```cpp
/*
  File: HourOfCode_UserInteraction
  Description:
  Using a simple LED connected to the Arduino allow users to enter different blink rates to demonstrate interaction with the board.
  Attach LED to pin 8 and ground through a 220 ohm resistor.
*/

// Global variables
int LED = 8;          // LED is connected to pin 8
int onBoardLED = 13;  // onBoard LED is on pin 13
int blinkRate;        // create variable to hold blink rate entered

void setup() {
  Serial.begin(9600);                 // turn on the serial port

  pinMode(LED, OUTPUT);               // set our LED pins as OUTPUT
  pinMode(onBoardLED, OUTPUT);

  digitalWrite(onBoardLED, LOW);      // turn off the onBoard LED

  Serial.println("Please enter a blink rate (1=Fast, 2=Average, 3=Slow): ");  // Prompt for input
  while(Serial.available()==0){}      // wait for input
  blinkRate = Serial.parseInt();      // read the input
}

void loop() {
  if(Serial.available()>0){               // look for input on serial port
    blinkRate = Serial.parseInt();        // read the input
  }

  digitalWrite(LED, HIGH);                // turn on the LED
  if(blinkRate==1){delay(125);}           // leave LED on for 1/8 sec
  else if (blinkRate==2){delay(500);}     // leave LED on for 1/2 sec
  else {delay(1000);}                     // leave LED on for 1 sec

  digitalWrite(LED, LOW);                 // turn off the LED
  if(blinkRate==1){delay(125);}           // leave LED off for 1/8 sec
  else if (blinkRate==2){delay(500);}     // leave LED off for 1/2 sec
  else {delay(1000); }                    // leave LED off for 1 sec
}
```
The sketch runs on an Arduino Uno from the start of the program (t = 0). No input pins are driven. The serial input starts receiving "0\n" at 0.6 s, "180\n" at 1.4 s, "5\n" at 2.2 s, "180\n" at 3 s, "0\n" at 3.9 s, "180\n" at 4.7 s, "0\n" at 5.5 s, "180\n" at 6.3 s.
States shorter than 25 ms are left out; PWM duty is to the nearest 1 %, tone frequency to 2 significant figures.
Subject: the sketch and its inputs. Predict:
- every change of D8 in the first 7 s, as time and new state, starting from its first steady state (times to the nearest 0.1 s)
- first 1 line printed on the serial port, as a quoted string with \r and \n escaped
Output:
0 s low; 1.4 s high; 2.4 s low; 3.4 s high; 4.4 s low; 5.4 s high; 6.4 s low
"Please enter a blink rate (1=Fast, 2=Average, 3=Slow): \r\n"
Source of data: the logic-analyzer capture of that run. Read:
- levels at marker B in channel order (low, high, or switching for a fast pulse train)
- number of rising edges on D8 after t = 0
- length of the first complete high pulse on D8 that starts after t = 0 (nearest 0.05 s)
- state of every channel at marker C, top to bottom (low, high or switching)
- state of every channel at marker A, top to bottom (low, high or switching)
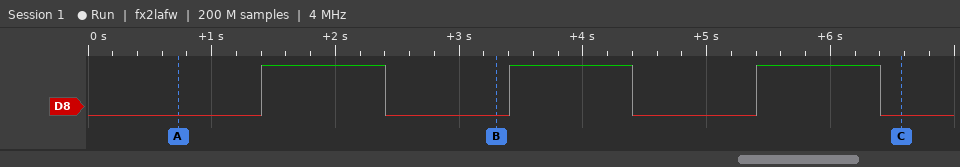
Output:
D8 low
3
1.00 s
D8 low
D8 low
